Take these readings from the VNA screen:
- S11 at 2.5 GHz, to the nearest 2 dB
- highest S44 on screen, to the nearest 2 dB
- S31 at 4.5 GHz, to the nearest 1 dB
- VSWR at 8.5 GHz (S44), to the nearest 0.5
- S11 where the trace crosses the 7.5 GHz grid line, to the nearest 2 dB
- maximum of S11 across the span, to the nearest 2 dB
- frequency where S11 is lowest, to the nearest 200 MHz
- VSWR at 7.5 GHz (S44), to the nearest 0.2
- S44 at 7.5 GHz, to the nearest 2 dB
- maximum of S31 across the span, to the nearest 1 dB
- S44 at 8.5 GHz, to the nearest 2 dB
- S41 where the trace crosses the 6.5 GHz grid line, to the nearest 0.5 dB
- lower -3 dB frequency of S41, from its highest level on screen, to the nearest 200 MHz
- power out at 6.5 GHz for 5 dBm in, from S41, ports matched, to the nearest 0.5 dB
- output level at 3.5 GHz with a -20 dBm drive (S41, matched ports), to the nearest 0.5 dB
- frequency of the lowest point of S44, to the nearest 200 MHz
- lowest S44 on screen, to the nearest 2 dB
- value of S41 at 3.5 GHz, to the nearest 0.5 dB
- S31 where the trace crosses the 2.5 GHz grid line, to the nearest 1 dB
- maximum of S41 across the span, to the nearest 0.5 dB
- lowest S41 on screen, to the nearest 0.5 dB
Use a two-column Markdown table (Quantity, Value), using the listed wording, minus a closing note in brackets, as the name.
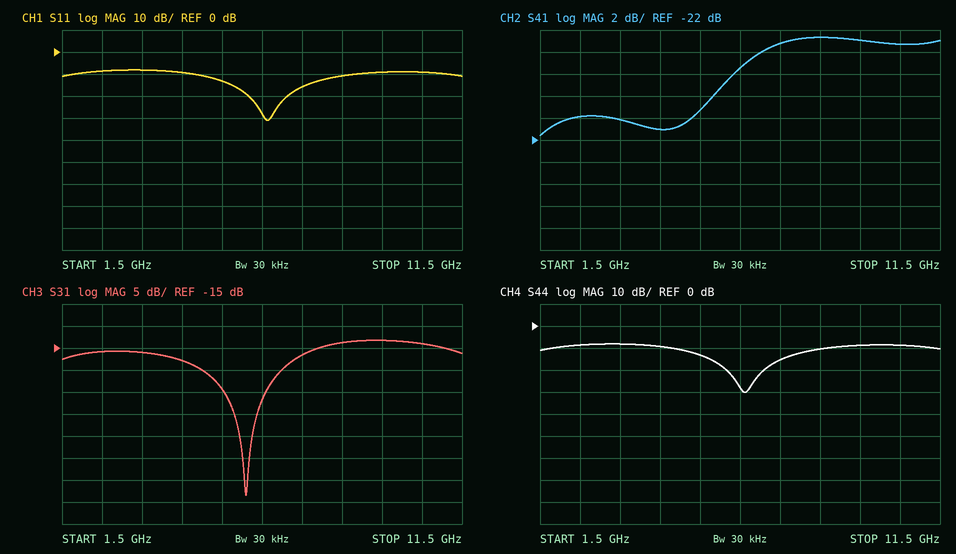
| Quantity | Value |
|---|---|
| S11 at 2.5 GHz, to the nearest 2 dB | -8 dB |
| highest S44 on screen, to the nearest 2 dB | -8 dB |
| S31 at 4.5 GHz, to the nearest 1 dB | -18 dB |
| VSWR at 8.5 GHz (S44), to the nearest 0.5 | 2.0 |
| S11 where the trace crosses the 7.5 GHz grid line, to the nearest 2 dB | -16 dB |
| maximum of S11 across the span, to the nearest 2 dB | -8 dB |
| frequency where S11 is lowest, to the nearest 200 MHz | 6.6 GHz |
| VSWR at 7.5 GHz (S44), to the nearest 0.2 | 1.4 |
| S44 at 7.5 GHz, to the nearest 2 dB | -16 dB |
| maximum of S31 across the span, to the nearest 1 dB | -13 dB |
| S44 at 8.5 GHz, to the nearest 2 dB | -10 dB |
| S41 where the trace crosses the 6.5 GHz grid line, to the nearest 0.5 dB | -15.5 dB |
| lower -3 dB frequency of S41, from its highest level on screen, to the nearest 200 MHz | 6.4 GHz |
| power out at 6.5 GHz for 5 dBm in, from S41, ports matched, to the nearest 0.5 dB | -10.5 dBm |
| output level at 3.5 GHz with a -20 dBm drive (S41, matched ports), to the nearest 0.5 dB | -40.0 dBm |
| frequency of the lowest point of S44, to the nearest 200 MHz | 6.6 GHz |
| lowest S44 on screen, to the nearest 2 dB | -30 dB |
| value of S41 at 3.5 GHz, to the nearest 0.5 dB | -20.0 dB |
| S31 where the trace crosses the 2.5 GHz grid line, to the nearest 1 dB | -16 dB |
| maximum of S41 across the span, to the nearest 0.5 dB | -12.5 dB |
| lowest S41 on screen, to the nearest 0.5 dB | -21.5 dB |
